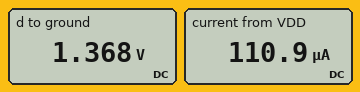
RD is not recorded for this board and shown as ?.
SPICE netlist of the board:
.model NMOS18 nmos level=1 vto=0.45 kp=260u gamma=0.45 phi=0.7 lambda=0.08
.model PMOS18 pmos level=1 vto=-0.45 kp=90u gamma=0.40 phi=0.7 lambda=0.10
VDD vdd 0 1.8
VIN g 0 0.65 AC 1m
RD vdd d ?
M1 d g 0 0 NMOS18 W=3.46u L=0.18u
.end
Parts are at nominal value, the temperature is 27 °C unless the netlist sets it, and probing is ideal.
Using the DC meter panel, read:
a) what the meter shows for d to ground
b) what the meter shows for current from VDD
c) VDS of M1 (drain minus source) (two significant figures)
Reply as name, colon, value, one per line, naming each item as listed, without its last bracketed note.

what the meter shows for d to ground: 1.368 V
what the meter shows for current from VDD: 110.9 µA
VDS of M1 (drain minus source): 1.4 V
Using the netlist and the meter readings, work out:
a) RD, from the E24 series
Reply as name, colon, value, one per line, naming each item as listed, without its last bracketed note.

RD, from the E24 series: 3.9 kΩ
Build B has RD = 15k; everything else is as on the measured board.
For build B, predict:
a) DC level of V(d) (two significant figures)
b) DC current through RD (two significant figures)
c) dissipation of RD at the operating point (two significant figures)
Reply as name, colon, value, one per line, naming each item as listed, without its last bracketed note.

DC level of V(d): 270 mV
DC current through RD: 100 µA
dissipation of RD at the operating point: 160 µW
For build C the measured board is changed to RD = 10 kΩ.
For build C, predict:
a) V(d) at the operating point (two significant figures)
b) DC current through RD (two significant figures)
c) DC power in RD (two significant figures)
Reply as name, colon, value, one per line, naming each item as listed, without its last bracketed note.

V(d) at the operating point: 740 mV
DC current through RD: 110 µA
DC power in RD: 110 µW
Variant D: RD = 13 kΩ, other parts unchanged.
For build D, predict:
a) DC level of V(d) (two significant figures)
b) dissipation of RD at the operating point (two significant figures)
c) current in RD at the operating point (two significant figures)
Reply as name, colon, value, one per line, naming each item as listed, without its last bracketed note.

DC level of V(d): 450 mV
dissipation of RD at the operating point: 140 µW
current in RD at the operating point: 100 µA
